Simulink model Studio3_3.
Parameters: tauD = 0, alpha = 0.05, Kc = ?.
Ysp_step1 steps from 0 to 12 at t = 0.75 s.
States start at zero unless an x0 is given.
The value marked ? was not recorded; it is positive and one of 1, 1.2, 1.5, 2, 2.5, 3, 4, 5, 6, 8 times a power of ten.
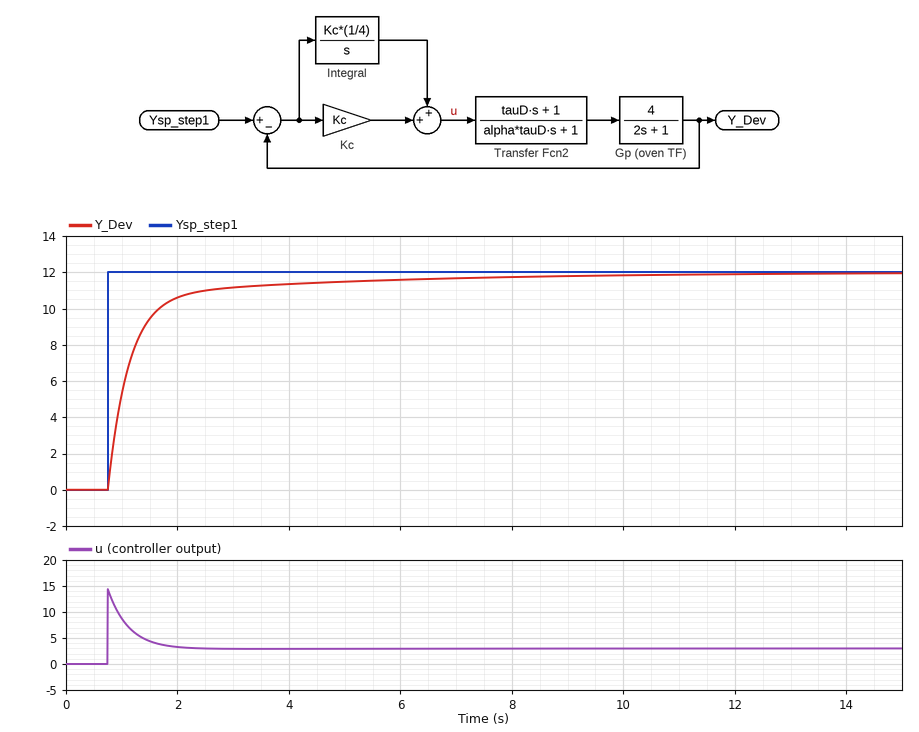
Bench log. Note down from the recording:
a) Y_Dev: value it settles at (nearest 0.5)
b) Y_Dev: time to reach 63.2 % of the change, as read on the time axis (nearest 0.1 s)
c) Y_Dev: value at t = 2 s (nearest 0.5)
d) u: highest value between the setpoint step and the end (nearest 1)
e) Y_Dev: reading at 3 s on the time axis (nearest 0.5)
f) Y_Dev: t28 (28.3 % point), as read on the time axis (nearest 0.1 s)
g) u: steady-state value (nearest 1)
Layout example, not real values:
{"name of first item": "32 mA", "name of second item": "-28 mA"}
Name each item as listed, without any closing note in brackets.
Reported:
{"Y_Dev: value it settles at": "12.0", "Y_Dev: time to reach 63.2 % of the change, as read on the time axis": "1.2 s", "Y_Dev: value at t = 2 s": "10.5", "u: highest value between the setpoint step and the end": "14", "Y_Dev: reading at 3 s on the time axis": "11.0", "Y_Dev: t28 (28.3 % point), as read on the time axis": "0.9 s", "u: steady-state value": "3"}
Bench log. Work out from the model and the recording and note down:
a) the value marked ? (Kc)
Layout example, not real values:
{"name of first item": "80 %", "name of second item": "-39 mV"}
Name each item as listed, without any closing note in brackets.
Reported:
{"the value marked ?": "1.2"}
